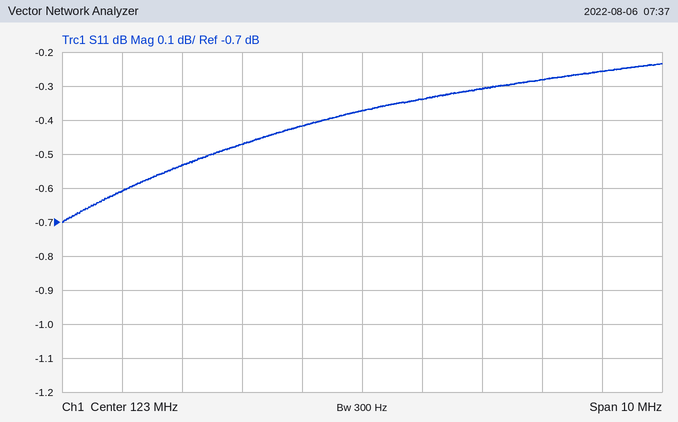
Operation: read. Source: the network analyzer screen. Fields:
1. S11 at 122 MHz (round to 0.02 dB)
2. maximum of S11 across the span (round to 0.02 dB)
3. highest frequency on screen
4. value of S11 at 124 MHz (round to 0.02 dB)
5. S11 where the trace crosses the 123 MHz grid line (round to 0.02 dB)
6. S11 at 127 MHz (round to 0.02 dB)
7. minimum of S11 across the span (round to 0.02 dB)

-0.42 dB
-0.24 dB
128 MHz
-0.34 dB
-0.38 dB
-0.26 dB
-0.70 dB
